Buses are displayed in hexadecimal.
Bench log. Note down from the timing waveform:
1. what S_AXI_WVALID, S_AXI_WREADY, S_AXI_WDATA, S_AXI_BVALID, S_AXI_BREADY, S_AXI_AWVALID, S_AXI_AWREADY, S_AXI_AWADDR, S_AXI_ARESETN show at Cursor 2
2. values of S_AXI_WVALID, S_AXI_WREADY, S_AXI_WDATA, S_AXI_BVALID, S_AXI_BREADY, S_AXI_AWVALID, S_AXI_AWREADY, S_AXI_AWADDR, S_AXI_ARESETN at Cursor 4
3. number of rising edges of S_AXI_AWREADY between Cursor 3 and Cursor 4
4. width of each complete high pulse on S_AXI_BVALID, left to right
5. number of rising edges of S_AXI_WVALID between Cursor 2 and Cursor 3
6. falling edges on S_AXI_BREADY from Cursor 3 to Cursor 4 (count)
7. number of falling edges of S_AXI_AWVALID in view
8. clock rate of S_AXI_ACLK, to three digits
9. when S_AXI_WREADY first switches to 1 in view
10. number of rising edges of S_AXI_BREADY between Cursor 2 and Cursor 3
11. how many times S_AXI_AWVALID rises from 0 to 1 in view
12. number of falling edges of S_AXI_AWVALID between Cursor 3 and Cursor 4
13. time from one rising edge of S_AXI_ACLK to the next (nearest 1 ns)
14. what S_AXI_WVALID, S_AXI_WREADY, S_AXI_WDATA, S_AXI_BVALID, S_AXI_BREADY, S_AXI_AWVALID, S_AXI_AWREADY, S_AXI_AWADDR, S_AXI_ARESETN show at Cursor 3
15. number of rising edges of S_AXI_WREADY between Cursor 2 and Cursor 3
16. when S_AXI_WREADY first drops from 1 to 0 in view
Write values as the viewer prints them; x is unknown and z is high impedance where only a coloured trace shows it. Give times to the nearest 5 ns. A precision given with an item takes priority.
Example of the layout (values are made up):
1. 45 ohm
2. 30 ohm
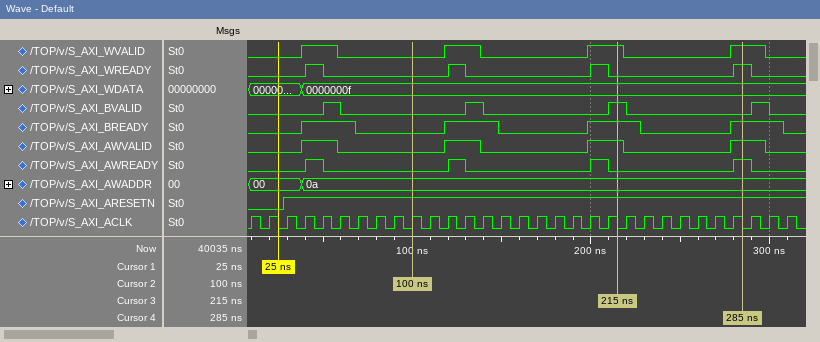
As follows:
1. S_AXI_WVALID=0, S_AXI_WREADY=0, S_AXI_WDATA=0000000f, S_AXI_BVALID=0, S_AXI_BREADY=0, S_AXI_AWVALID=0, S_AXI_AWREADY=0, S_AXI_AWADDR=0a, S_AXI_ARESETN=1
2. S_AXI_WVALID=1, S_AXI_WREADY=1, S_AXI_WDATA=0000000f, S_AXI_BVALID=0, S_AXI_BREADY=1, S_AXI_AWVALID=1, S_AXI_AWREADY=1, S_AXI_AWADDR=0a, S_AXI_ARESETN=1
3. 1
4. 10 ns, 10 ns, 10 ns, 10 ns
5. 2
6. 1
7. 4
8. 100 MHz
9. 40 ns
10. 2
11. 4
12. 1
13. 10 ns
14. S_AXI_WVALID=1, S_AXI_WREADY=0, S_AXI_WDATA=0000000f, S_AXI_BVALID=1, S_AXI_BREADY=1, S_AXI_AWVALID=1, S_AXI_AWREADY=0, S_AXI_AWADDR=0a, S_AXI_ARESETN=1
15. 2
16. 50 ns
